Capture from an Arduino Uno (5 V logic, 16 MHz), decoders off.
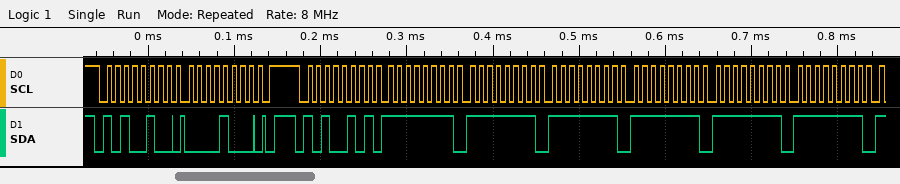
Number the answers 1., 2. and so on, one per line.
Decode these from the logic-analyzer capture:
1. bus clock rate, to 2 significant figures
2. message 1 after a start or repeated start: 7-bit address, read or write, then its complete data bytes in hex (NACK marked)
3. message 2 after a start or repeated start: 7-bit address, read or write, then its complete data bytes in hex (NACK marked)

1. 100 kHz
2. 0x52 write: 08
3. 0x52 read: FF FF FF FF FF FF
